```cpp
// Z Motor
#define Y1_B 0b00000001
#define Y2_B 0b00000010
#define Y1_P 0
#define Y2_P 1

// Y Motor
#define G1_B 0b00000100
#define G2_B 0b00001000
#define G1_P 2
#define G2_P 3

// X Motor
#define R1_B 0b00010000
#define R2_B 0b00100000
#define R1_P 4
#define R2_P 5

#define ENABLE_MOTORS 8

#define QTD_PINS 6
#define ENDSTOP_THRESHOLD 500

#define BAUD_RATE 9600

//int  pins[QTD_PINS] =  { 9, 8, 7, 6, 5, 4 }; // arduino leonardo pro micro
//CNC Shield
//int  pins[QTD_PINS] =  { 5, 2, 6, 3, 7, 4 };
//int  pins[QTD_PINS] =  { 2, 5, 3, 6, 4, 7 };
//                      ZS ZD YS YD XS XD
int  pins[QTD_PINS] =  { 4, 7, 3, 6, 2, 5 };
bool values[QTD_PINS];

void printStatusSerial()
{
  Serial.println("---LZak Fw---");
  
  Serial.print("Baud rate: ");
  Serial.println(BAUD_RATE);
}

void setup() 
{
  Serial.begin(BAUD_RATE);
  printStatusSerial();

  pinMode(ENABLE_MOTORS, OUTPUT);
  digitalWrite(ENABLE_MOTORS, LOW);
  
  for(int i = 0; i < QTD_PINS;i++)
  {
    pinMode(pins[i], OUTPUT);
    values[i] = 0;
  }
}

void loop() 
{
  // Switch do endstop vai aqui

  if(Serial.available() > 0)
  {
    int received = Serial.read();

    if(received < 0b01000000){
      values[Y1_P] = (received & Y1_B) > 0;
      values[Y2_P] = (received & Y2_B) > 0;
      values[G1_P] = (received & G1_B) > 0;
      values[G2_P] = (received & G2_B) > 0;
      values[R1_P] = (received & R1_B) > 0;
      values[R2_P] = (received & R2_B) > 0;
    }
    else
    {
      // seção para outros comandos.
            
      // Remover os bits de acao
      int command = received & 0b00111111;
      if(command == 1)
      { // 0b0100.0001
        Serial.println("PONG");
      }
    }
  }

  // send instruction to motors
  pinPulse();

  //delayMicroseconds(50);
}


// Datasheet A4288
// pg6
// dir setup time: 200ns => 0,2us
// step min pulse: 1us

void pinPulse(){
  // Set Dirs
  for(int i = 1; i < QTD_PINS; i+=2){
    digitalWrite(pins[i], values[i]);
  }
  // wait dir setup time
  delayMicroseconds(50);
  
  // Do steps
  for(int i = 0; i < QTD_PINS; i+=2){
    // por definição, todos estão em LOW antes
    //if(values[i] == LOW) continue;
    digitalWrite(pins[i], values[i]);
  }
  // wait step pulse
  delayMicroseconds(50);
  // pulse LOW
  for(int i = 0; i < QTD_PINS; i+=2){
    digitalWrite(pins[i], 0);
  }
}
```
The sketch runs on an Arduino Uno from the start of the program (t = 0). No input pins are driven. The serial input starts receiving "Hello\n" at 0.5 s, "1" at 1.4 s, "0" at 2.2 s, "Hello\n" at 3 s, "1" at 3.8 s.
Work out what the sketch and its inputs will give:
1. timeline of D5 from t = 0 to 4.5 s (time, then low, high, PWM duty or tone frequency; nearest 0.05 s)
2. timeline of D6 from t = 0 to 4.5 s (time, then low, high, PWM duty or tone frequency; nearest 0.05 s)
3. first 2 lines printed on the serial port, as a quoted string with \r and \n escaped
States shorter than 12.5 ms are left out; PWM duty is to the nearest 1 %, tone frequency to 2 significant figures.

0 s low; 1.4 s high; 3 s low; 3.8 s high
0 s low; 0.5 s high; 1.4 s low; 3 s high; 3.8 s low
"---LZak Fw---\r\nBaud rate: 9600\r\n"
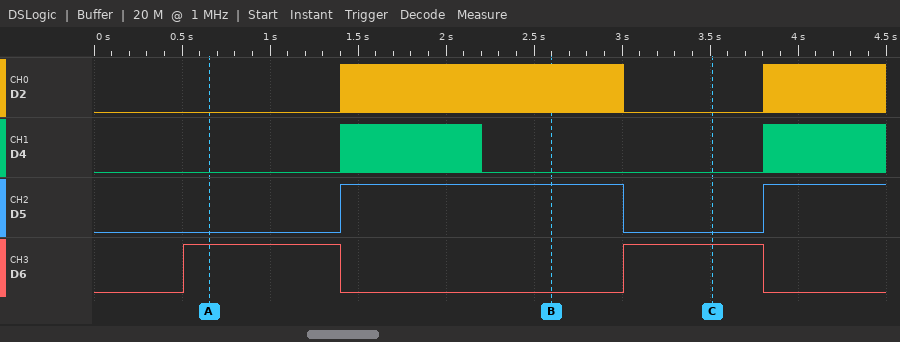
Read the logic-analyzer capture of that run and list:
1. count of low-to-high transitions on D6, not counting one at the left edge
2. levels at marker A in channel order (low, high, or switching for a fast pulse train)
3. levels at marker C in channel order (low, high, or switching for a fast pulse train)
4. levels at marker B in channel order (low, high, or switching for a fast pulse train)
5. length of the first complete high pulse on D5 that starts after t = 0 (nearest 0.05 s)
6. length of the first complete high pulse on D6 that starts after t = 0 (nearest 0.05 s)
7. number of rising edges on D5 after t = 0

2
D2 low, D4 low, D5 low, D6 high
D2 low, D4 low, D5 low, D6 high
D2 switching, D4 low, D5 high, D6 low
1.60 s
0.90 s
2
